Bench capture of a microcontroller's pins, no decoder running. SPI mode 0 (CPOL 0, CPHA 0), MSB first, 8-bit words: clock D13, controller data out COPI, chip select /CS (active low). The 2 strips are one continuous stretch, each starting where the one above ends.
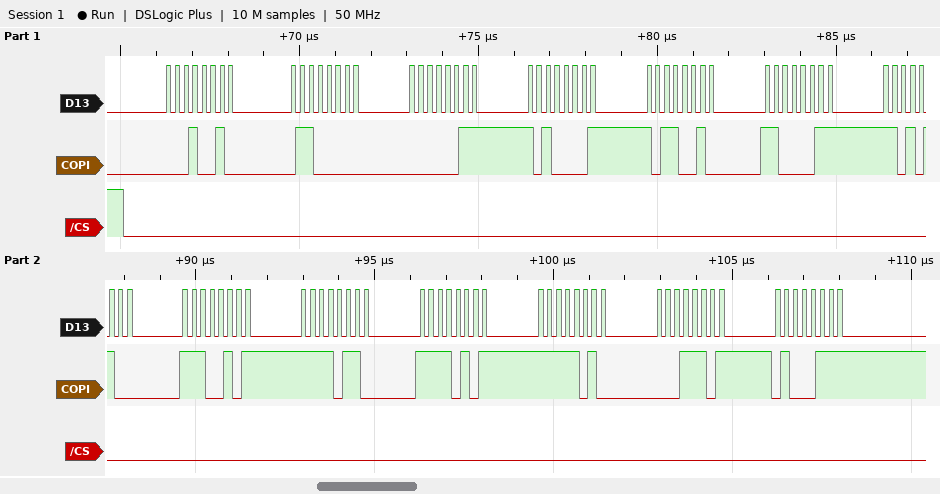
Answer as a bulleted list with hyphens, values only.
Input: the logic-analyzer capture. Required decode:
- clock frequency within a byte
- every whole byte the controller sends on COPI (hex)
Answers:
- 4 MHz
- 0x12 0x60 0x03 0xA1 0xB2 0xC3 0xD4 0xE5 0xF6 0xF5 0xFA 0x1D 0x47
